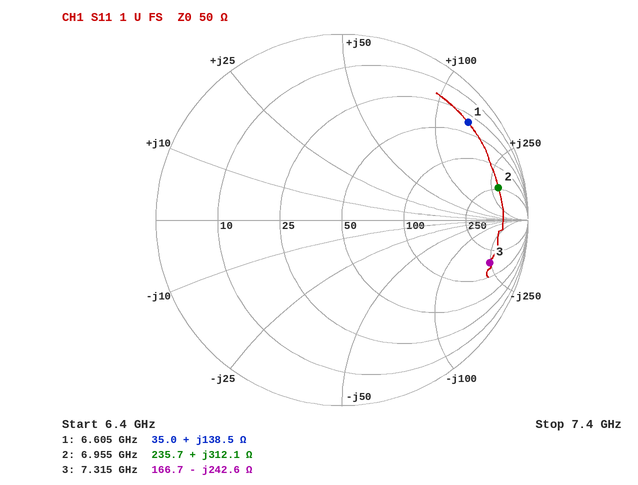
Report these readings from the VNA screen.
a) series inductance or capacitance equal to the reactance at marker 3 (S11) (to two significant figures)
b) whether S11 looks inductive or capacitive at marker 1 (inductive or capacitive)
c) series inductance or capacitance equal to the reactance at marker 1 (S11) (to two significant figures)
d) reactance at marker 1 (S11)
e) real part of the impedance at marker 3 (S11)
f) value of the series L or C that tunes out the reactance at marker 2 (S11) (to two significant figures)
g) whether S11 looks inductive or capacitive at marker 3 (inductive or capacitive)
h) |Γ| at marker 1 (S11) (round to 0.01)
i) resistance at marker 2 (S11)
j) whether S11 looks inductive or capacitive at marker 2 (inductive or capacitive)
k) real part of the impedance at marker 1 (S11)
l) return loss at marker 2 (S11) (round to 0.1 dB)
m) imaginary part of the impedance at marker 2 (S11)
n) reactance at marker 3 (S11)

90 fF
inductive
3.3 nH
+138.5 Ω
166.7 Ω
73 fF
capacitive
0.86
235.7 Ω
inductive
35.0 Ω
1.3 dB
+312.1 Ω
-242.6 Ω
